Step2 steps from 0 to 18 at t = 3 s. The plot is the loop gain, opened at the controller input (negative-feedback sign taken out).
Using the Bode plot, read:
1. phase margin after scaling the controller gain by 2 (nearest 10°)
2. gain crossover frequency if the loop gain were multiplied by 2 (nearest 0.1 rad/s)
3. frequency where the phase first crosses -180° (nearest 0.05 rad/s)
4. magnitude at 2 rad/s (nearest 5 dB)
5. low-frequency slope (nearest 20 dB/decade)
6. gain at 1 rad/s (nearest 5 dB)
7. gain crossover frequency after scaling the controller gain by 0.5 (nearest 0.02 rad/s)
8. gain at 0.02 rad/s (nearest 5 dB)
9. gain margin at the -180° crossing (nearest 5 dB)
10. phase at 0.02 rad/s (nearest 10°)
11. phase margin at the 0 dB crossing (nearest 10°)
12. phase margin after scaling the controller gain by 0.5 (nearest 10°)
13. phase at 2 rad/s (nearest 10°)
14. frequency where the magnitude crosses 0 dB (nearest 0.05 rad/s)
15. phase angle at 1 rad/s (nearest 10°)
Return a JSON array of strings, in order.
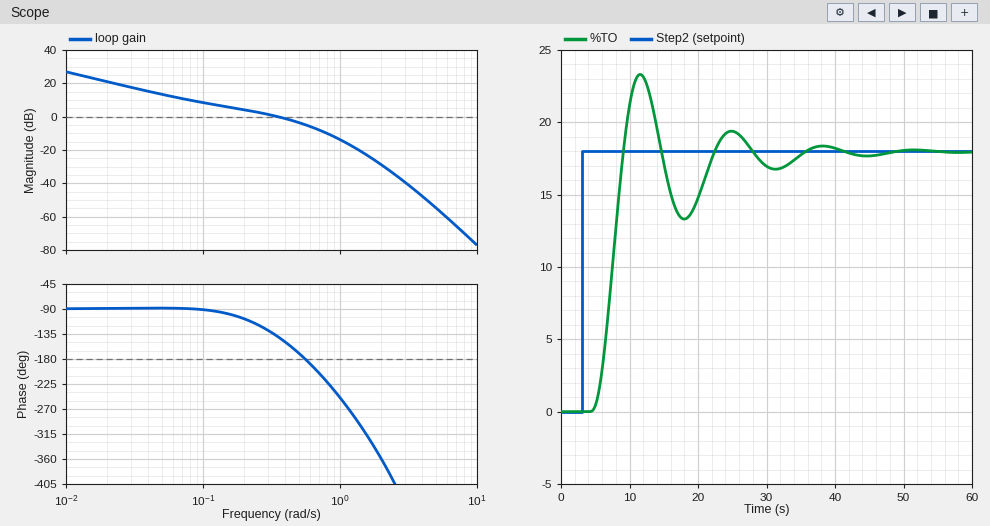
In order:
["-10°", "0.6 rad/s", "0.55 rad/s", "-30 dB", "-20 dB/decade", "-15 dB", "0.14 rad/s", "20 dB", "5 dB", "-90°", "40°", "80°", "-360°", "0.35 rad/s", "-250°"]
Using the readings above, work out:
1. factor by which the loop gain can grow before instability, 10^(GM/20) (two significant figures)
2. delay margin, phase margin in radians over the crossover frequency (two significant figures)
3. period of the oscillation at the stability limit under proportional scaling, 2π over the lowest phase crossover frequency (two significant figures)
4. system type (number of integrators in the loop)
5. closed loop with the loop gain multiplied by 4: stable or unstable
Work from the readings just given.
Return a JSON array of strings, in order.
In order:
["1.8", "2.0 s", "11 s", "1", "unstable"]
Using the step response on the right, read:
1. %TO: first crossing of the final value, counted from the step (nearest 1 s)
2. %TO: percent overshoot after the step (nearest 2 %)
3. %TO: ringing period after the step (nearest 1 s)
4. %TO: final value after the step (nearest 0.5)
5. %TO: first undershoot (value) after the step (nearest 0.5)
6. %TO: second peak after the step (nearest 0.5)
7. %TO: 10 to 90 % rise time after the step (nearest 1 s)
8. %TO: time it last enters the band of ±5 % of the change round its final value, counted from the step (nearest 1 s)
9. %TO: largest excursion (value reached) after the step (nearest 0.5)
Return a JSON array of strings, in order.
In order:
["6 s", "30 %", "13 s", "18.0", "13.5", "19.5", "3 s", "30 s", "23.5"]
